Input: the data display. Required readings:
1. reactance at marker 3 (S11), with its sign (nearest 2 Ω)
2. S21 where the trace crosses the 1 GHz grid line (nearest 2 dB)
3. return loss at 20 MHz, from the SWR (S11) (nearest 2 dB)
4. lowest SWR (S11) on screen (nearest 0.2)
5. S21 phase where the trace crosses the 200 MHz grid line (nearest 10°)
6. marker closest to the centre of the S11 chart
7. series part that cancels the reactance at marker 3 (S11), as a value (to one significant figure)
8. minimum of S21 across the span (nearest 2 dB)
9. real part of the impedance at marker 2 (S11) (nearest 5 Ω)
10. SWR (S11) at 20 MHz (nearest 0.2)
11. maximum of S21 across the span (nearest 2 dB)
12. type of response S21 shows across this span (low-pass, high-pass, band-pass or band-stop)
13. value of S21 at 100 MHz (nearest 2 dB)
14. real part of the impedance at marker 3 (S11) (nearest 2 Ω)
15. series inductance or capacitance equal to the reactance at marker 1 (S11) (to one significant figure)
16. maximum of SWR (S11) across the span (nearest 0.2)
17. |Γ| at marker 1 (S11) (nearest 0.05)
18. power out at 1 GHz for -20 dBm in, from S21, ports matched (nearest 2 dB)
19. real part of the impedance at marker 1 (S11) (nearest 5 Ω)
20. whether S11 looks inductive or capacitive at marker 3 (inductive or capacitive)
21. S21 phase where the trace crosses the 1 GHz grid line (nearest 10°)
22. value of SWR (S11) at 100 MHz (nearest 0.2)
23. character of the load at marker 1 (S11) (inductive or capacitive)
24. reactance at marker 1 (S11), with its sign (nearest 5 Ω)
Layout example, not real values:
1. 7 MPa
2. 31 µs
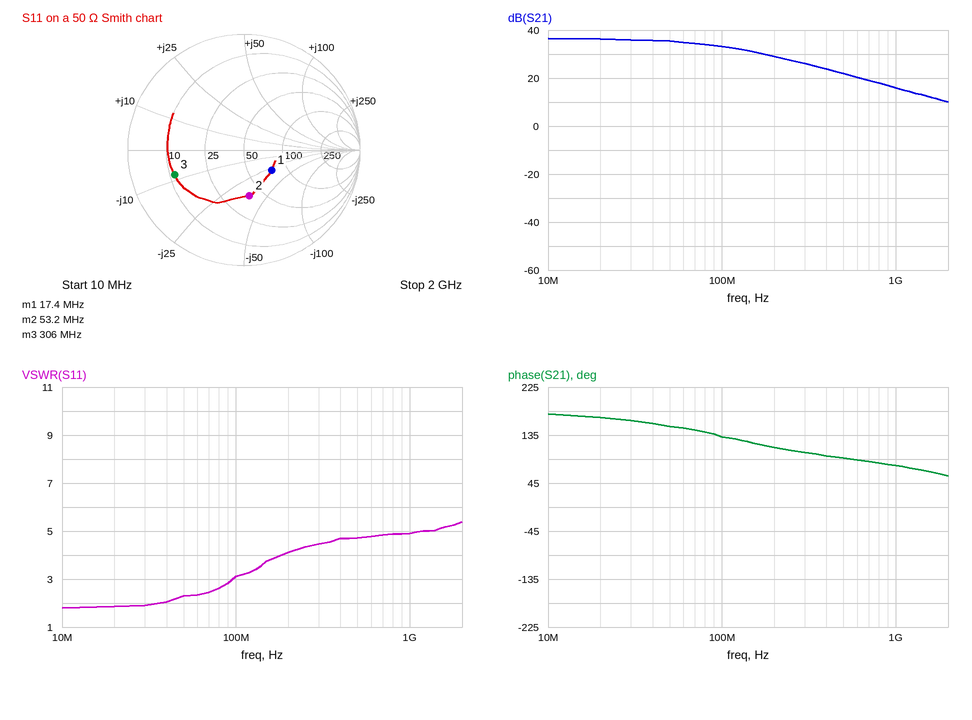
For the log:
1. -8 Ω
2. 16 dB
3. 10 dB
4. 1.8
5. 110°
6. marker 1
7. 4 nH
8. 10 dB
9. 40 Ω
10. 1.8
11. 36 dB
12. low-pass
13. 34 dB
14. 12 Ω
15. 300 pF
16. 5.4
17. 0.30
18. -4 dBm
19. 75 Ω
20. capacitive
21. 80°
22. 3.2
23. capacitive
24. -30 Ω
